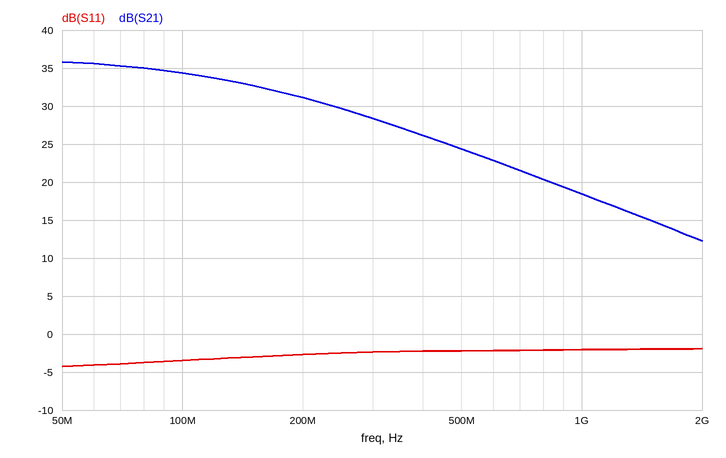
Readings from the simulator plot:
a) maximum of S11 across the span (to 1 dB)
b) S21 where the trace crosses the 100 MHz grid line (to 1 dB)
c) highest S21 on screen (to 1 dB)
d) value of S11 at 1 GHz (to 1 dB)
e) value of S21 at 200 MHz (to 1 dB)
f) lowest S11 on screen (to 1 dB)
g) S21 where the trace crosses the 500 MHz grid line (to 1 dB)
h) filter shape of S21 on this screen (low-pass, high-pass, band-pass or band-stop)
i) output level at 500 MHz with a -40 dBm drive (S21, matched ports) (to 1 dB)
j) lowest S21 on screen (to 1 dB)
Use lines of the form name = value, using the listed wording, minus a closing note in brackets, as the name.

maximum of S11 across the span = -2 dB
S21 where the trace crosses the 100 MHz grid line = 34 dB
highest S21 on screen = 36 dB
value of S11 at 1 GHz = -2 dB
value of S21 at 200 MHz = 31 dB
lowest S11 on screen = -4 dB
S21 where the trace crosses the 500 MHz grid line = 24 dB
filter shape of S21 on this screen = low-pass
output level at 500 MHz with a -40 dBm drive (S21, matched ports) = -16 dBm
lowest S21 on screen = 12 dB
